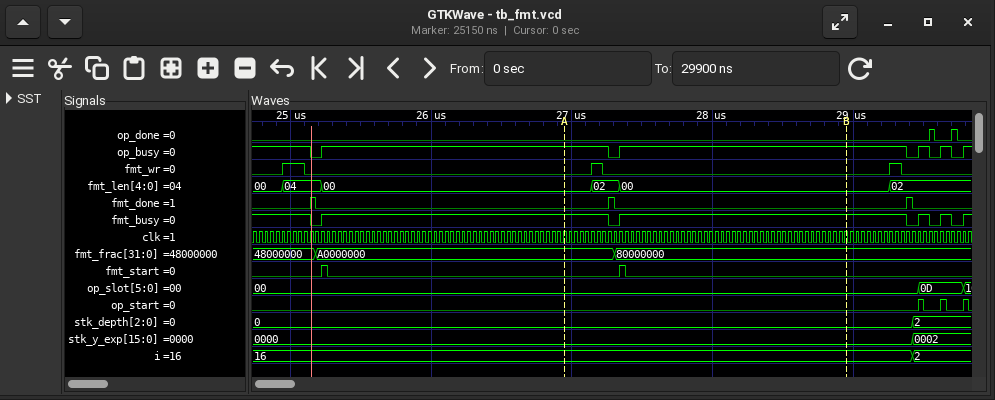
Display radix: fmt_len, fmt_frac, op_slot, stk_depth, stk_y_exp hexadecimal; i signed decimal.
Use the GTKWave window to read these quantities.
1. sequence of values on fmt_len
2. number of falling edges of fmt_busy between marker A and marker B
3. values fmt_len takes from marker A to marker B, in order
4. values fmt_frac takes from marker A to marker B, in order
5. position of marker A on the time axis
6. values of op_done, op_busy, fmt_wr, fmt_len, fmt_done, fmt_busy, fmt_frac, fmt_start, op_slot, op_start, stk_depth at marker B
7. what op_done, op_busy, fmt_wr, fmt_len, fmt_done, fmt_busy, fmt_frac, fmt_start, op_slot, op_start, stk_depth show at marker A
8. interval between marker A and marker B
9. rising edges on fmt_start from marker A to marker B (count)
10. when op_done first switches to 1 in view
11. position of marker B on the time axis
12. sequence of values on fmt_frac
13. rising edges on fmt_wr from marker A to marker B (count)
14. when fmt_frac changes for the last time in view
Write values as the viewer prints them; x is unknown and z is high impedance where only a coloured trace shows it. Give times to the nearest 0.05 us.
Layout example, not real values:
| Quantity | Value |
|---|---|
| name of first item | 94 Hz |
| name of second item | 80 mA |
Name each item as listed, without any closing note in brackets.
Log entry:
| Quantity | Value |
|---|---|
| sequence of values on fmt_len | 00, 04, 00, 02, 00, 02 |
| number of falling edges of fmt_busy between marker A and marker B | 1 |
| values fmt_len takes from marker A to marker B, in order | 00, 02, 00 |
| values fmt_frac takes from marker A to marker B, in order | A0000000, 80000000 |
| position of marker A on the time axis | 26.95 us |
| values of op_done, op_busy, fmt_wr, fmt_len, fmt_done, fmt_busy, fmt_frac, fmt_start, op_slot, op_start, stk_depth at marker B | op_done=0, op_busy=1, fmt_wr=0, fmt_len=00, fmt_done=0, fmt_busy=1, fmt_frac=80000000, fmt_start=0, op_slot=00, op_start=0, stk_depth=0 |
| what op_done, op_busy, fmt_wr, fmt_len, fmt_done, fmt_busy, fmt_frac, fmt_start, op_slot, op_start, stk_depth show at marker A | op_done=0, op_busy=1, fmt_wr=0, fmt_len=00, fmt_done=0, fmt_busy=1, fmt_frac=A0000000, fmt_start=0, op_slot=00, op_start=0, stk_depth=0 |
| interval between marker A and marker B | 2 us |
| rising edges on fmt_start from marker A to marker B | 1 |
| when op_done first switches to 1 in view | 29.55 us |
| position of marker B on the time axis | 28.95 us |
| sequence of values on fmt_frac | 48000000, A0000000, 80000000 |
| rising edges on fmt_wr from marker A to marker B | 1 |
| when fmt_frac changes for the last time in view | 27.3 us |
